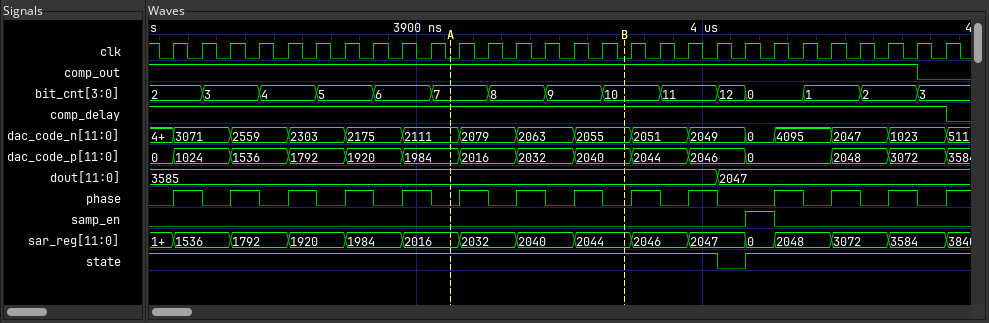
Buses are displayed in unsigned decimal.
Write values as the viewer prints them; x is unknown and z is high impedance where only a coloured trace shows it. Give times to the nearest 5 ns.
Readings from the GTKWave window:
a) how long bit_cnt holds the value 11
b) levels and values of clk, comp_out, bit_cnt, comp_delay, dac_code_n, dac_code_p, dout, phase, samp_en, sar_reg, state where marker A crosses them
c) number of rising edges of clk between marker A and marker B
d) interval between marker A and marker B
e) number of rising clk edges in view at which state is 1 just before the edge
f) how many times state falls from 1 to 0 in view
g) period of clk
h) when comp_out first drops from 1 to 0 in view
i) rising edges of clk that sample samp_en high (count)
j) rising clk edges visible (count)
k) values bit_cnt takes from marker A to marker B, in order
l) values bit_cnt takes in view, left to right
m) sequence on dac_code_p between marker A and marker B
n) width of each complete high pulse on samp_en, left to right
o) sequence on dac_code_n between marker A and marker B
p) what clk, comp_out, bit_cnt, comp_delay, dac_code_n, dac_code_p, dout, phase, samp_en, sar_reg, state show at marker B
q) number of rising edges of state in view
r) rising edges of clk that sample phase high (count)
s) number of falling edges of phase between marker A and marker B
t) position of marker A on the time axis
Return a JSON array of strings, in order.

["20 ns", "clk=0, comp_out=1, bit_cnt=7, comp_delay=1, dac_code_n=2111, dac_code_p=1984, dout=3585, phase=0, samp_en=0, sar_reg=2016, state=1", "6", "60 ns", "27", "1", "10 ns", "4075 ns", "1", "28", "7, 8, 9, 10", "2, 3, 4, 5, 6, 7, 8, 9, 10, 11, 12, 0, 1, 2, 3", "1984, 2016, 2032, 2040", "10 ns", "2111, 2079, 2063, 2055", "clk=0, comp_out=1, bit_cnt=10, comp_delay=1, dac_code_n=2055, dac_code_p=2040, dout=3585, phase=0, samp_en=0, sar_reg=2044, state=1", "1", "13", "3", "3910 ns"]
